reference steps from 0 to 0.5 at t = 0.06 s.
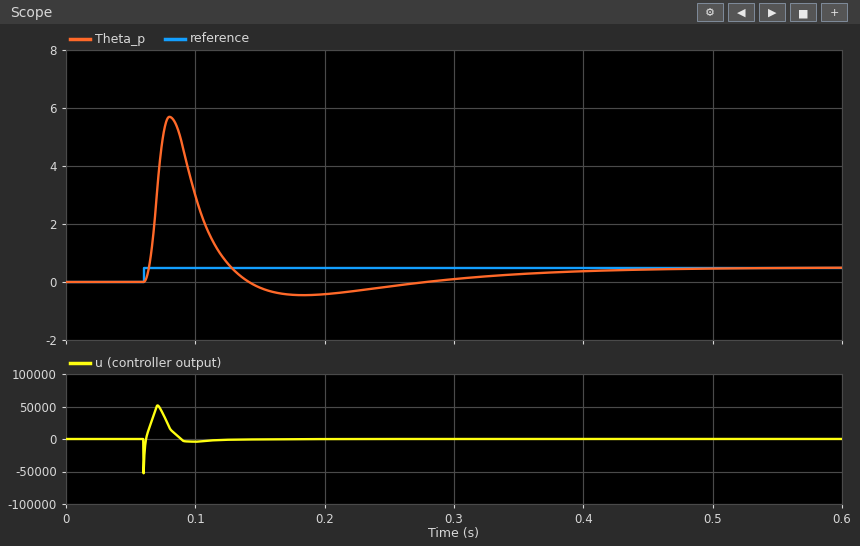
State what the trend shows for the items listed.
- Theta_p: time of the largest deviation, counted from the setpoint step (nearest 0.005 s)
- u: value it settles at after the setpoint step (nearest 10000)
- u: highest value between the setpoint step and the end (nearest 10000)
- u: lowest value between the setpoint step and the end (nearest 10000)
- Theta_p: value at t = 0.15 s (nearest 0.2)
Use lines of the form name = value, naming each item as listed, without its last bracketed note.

Theta_p: time of the largest deviation, counted from the setpoint step = 0.020 s
u: value it settles at after the setpoint step = 0
u: highest value between the setpoint step and the end = 50000
u: lowest value between the setpoint step and the end = -50000
Theta_p: value at t = 0.15 s = -0.2
